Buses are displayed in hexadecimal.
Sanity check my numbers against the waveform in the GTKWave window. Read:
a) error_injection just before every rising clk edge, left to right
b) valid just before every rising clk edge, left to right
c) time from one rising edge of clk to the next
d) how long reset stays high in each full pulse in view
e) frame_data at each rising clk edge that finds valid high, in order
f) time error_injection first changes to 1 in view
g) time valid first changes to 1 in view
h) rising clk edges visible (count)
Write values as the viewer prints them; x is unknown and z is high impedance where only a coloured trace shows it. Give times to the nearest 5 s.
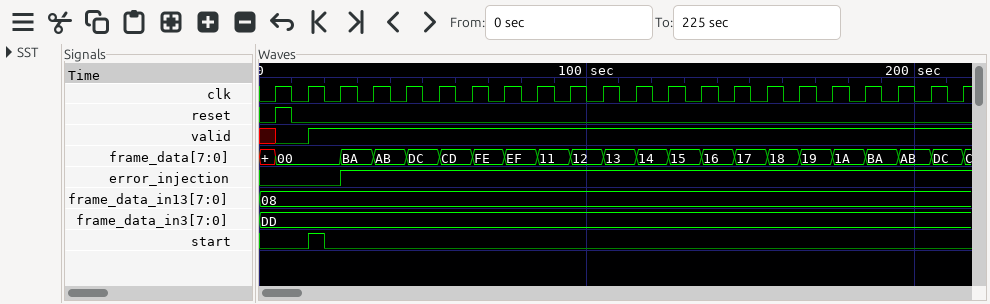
0 0 0 1 1 1 1 1 1 1 1 1 1 1 1 1 1 1 1 1 1 1
x 0 1 1 1 1 1 1 1 1 1 1 1 1 1 1 1 1 1 1 1 1
10 s
5 s
00, BA, AB, DC, CD, FE, EF, 11, 12, 13, 14, 15, 16, 17, 18, 19, 1A, BA, AB, DC
25 s
15 s
22
